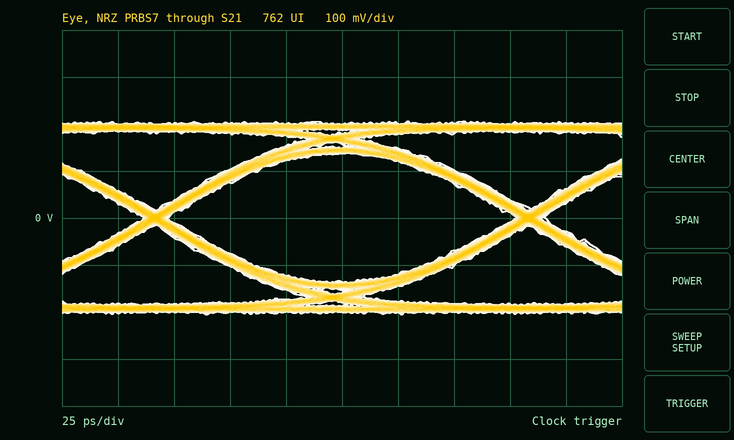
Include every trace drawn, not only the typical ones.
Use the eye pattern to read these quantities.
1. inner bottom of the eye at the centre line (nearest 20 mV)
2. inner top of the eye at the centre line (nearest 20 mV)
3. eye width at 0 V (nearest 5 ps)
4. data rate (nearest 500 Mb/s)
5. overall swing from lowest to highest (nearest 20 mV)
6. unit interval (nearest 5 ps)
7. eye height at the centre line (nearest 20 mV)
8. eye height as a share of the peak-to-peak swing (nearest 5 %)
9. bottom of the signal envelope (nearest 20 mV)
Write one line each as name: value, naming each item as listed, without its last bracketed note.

inner bottom of the eye at the centre line: -140 mV
inner top of the eye at the centre line: 140 mV
eye width at 0 V: 155 ps
data rate: 6.0 Gb/s
overall swing from lowest to highest: 420 mV
unit interval: 165 ps
eye height at the centre line: 280 mV
eye height as a share of the peak-to-peak swing: 65 %
bottom of the signal envelope: -200 mV
